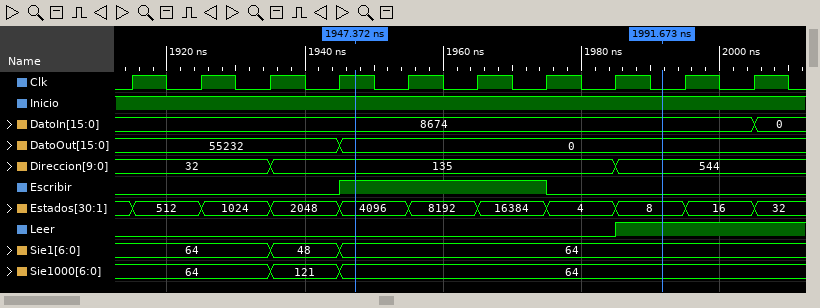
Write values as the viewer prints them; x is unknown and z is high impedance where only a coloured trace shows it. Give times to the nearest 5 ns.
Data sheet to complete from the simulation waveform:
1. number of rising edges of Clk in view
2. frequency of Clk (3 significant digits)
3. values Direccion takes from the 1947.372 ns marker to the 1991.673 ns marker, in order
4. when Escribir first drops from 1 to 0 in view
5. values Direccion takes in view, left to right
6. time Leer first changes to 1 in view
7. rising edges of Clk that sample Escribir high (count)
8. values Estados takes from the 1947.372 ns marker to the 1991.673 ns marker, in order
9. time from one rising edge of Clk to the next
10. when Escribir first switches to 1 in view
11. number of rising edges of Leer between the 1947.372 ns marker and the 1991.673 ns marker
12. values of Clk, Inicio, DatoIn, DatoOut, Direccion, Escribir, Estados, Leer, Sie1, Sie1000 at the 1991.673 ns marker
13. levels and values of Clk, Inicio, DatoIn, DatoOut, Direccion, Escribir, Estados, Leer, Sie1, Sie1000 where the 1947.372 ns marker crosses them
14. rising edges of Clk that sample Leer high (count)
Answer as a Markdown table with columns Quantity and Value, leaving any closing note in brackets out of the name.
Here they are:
| Quantity | Value |
|---|---|
| number of rising edges of Clk in view | 10 |
| frequency of Clk | 100 MHz |
| values Direccion takes from the 1947.372 ns marker to the 1991.673 ns marker, in order | 135, 544 |
| when Escribir first drops from 1 to 0 in view | 1975 ns |
| values Direccion takes in view, left to right | 32, 135, 544 |
| time Leer first changes to 1 in view | 1985 ns |
| rising edges of Clk that sample Escribir high | 3 |
| values Estados takes from the 1947.372 ns marker to the 1991.673 ns marker, in order | 4096, 8192, 16384, 4, 8 |
| time from one rising edge of Clk to the next | 10 ns |
| when Escribir first switches to 1 in view | 1945 ns |
| number of rising edges of Leer between the 1947.372 ns marker and the 1991.673 ns marker | 1 |
| values of Clk, Inicio, DatoIn, DatoOut, Direccion, Escribir, Estados, Leer, Sie1, Sie1000 at the 1991.673 ns marker | Clk=0, Inicio=1, DatoIn=8674, DatoOut=0, Direccion=544, Escribir=0, Estados=8, Leer=1, Sie1=64, Sie1000=64 |
| levels and values of Clk, Inicio, DatoIn, DatoOut, Direccion, Escribir, Estados, Leer, Sie1, Sie1000 where the 1947.372 ns marker crosses them | Clk=1, Inicio=1, DatoIn=8674, DatoOut=0, Direccion=135, Escribir=1, Estados=4096, Leer=0, Sie1=64, Sie1000=64 |
| rising edges of Clk that sample Leer high | 2 |
